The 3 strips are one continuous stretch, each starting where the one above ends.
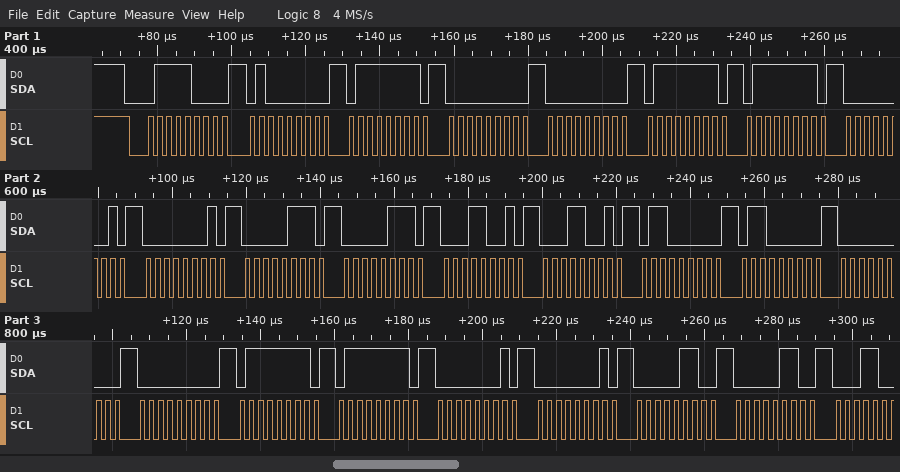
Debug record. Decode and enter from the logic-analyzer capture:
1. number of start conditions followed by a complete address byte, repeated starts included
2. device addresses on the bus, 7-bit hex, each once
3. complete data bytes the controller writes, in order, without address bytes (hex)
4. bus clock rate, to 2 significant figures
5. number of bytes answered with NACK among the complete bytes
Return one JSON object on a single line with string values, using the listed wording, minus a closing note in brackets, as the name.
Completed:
{"number of start conditions followed by a complete address byte, repeated starts included": "1", "device addresses on the bus, 7-bit hex, each once": "0x3C", "complete data bytes the controller writes, in order, without address bytes": "40 7F 00 00 7F 7F 01 01 07 07 19 19 60 60 00 00 7F 7F 01 01 06 06", "bus clock rate, to 2 significant figures": "400 kHz", "number of bytes answered with NACK among the complete bytes": "0"}
